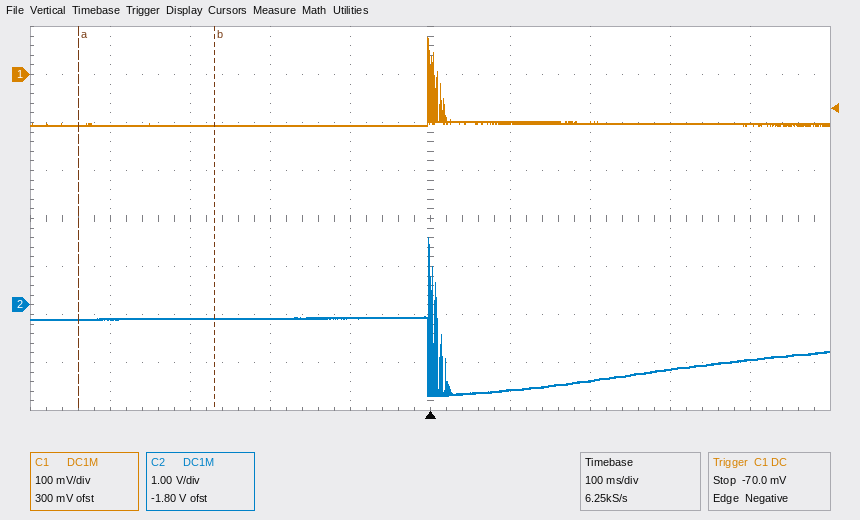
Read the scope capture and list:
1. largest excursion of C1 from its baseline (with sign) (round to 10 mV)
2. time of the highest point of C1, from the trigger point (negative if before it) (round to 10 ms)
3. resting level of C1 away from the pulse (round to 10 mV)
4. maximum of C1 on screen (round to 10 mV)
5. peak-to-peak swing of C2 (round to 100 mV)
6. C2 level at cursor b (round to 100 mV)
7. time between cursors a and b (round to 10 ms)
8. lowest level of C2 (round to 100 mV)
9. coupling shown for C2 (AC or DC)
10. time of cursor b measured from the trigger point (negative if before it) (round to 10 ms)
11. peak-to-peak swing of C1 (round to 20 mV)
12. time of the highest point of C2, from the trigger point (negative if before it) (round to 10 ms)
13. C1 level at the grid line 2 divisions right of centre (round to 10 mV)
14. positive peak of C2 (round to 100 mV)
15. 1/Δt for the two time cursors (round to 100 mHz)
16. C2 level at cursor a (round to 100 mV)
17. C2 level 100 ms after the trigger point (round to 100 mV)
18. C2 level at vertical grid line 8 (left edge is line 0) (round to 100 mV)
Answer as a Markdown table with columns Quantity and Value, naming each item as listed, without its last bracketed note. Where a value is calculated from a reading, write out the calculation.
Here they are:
| Quantity | Value |
|---|---|
| largest excursion of C1 from its baseline (with sign) | 80 mV − (-100 mV) = +180 mV |
| time of the highest point of C1, from the trigger point (negative if before it) | 0 ms |
| resting level of C1 away from the pulse | -100 mV |
| maximum of C1 on screen | 80 mV |
| peak-to-peak swing of C2 | 1.4 V − (-1.9 V) = 3.3 V |
| C2 level at cursor b | -300 mV |
| time between cursors a and b | 170 ms |
| lowest level of C2 | -1.9 V |
| coupling shown for C2 | DC |
| time of cursor b measured from the trigger point (negative if before it) | -270 ms |
| peak-to-peak swing of C1 | 180 mV |
| time of the highest point of C2, from the trigger point (negative if before it) | 0 ms |
| C1 level at the grid line 2 divisions right of centre | -100 mV |
| positive peak of C2 | 1.4 V |
| 1/Δt for the two time cursors | 1 / 170 ms ≈ 5.9 Hz |
| C2 level at cursor a | -300 mV |
| C2 level 100 ms after the trigger point | -1.8 V |
| C2 level at vertical grid line 8 (left edge is line 0) | -1.3 V |
